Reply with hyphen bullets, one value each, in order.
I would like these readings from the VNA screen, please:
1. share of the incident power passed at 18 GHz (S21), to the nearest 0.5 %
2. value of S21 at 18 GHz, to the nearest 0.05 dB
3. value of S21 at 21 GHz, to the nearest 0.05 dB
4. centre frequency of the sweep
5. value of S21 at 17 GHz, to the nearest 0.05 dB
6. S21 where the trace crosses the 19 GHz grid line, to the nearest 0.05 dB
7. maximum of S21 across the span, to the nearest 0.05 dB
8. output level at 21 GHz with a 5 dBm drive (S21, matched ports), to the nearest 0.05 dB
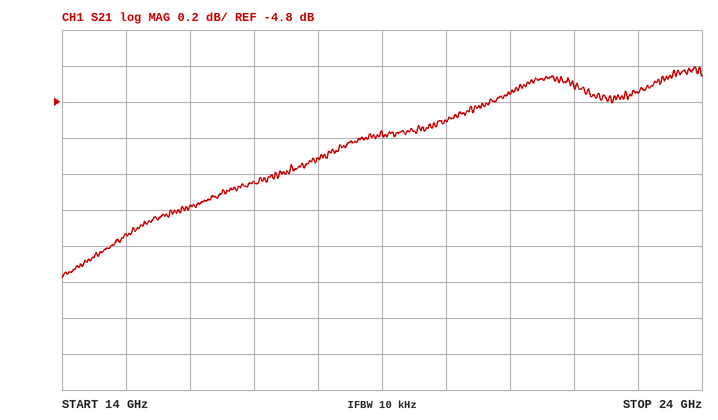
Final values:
- 31.0 %
- -5.10 dB
- -4.75 dB
- 19 GHz
- -5.25 dB
- -4.95 dB
- -4.60 dB
- 0.25 dBm
